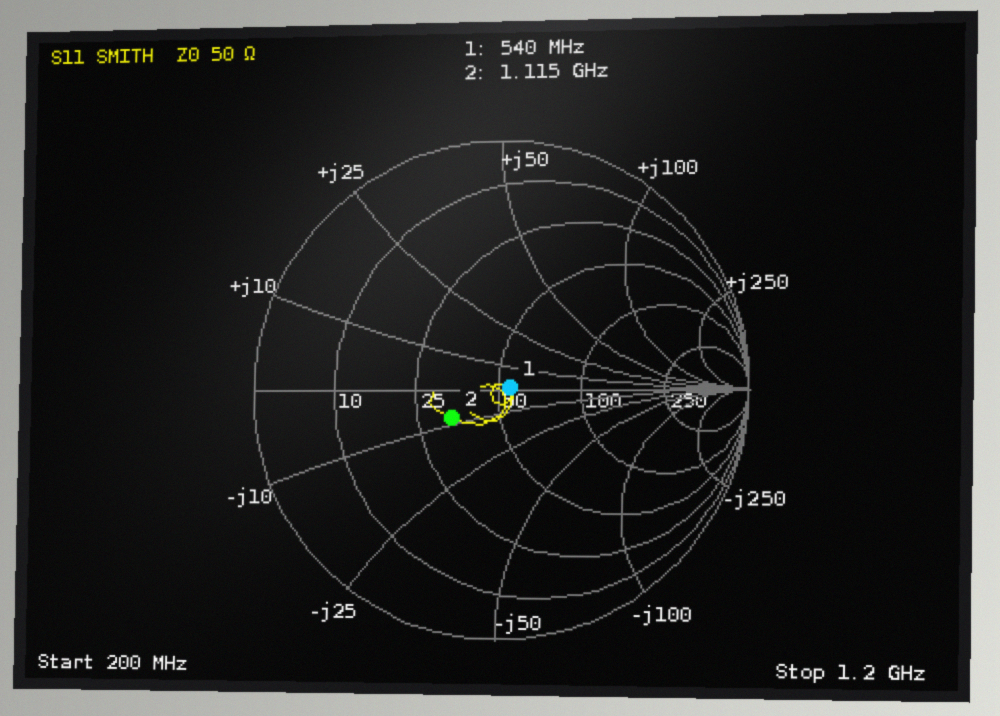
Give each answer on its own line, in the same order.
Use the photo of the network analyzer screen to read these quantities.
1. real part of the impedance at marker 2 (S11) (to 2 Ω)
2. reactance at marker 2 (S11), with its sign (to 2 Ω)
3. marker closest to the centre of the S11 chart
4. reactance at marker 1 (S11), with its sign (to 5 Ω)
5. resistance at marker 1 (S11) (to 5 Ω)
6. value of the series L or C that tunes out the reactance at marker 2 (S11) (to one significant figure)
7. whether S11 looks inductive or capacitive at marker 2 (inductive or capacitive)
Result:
34 Ω
-8 Ω
marker 1
0 Ω
55 Ω
1 nH
capacitive
